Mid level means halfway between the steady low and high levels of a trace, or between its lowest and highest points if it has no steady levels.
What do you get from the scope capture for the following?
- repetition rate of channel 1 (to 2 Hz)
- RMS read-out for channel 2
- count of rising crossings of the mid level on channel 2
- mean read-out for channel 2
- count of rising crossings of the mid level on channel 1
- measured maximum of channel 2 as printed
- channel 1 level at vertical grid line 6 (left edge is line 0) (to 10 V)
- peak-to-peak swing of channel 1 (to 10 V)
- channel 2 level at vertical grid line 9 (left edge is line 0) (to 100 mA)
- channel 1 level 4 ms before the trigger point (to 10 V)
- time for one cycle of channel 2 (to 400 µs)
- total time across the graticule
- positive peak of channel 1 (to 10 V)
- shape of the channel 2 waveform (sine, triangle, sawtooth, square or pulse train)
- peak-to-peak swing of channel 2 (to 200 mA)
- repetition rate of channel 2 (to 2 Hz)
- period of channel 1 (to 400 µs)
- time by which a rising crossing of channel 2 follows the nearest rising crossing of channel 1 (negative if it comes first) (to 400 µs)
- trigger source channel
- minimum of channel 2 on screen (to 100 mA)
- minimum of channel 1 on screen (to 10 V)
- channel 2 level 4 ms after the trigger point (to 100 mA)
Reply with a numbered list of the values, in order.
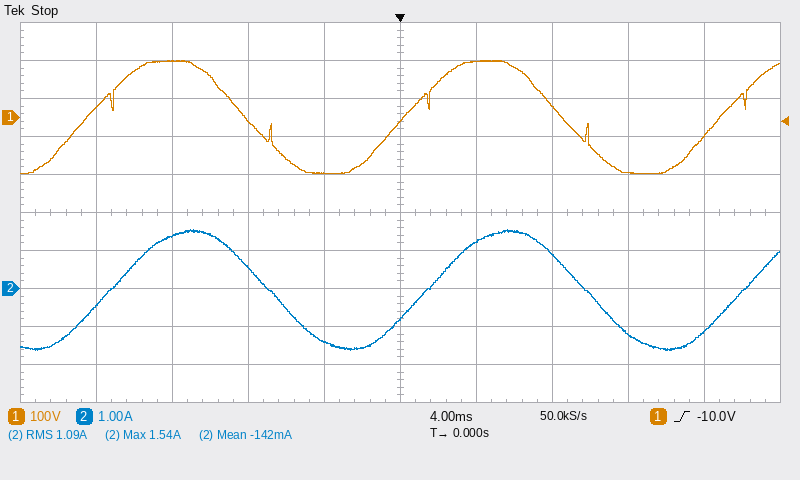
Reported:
1. 60 Hz
2. 1.09 A
3. 3
4. -142 mA
5. 3
6. 1.54 A
7. 150 V
8. 300 V
9. -1.1 A
10. -150 V
11. 16.8 ms
12. 40 ms
13. 150 V
14. sine
15. 3.2 A
16. 60 Hz
17. 16.8 ms
18. +1.2 ms
19. channel 1
20. -1.6 A
21. -150 V
22. 1.2 A
